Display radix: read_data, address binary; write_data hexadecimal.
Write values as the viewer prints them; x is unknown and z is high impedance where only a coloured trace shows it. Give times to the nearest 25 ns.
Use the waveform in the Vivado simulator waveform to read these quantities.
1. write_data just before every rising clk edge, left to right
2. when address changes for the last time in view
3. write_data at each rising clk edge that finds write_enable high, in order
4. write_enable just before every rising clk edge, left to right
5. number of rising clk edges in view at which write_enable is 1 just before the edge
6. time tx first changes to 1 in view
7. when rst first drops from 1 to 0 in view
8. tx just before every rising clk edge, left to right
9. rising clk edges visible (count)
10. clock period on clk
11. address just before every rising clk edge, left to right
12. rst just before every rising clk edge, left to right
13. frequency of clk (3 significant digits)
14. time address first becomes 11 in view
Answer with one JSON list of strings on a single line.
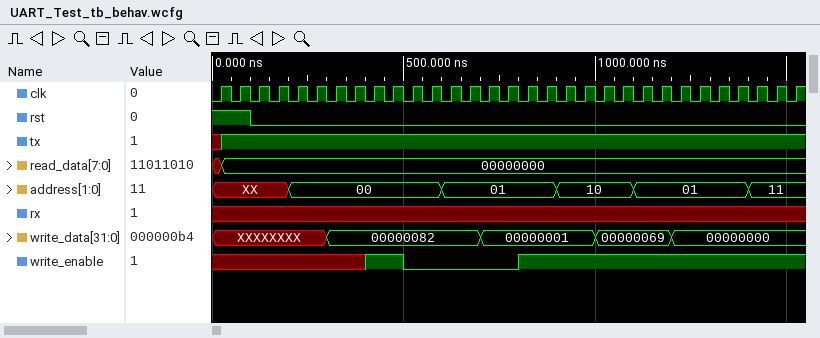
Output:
["XXXXXXXX, XXXXXXXX, XXXXXXXX, XXXXXXXX, XXXXXXXX, XXXXXXXX, 00000082, 00000082, 00000082, 00000082, 00000082, 00000082, 00000082, 00000082, 00000001, 00000001, 00000001, 00000001, 00000001, 00000001, 00000069, 00000069, 00000069, 00000069, 00000000, 00000000, 00000000, 00000000, 00000000, 00000000, 00000000", "1400 ns", "00000082, 00000082, 00000001, 00000001, 00000001, 00000001, 00000069, 00000069, 00000069, 00000069, 00000000, 00000000, 00000000, 00000000, 00000000, 00000000, 00000000", "x x x x x x x x 1 1 0 0 0 0 0 0 1 1 1 1 1 1 1 1 1 1 1 1 1 1 1", "17", "25 ns", "100 ns", "x 1 1 1 1 1 1 1 1 1 1 1 1 1 1 1 1 1 1 1 1 1 1 1 1 1 1 1 1 1 1", "31", "50 ns", "XX, XX, XX, XX, 00, 00, 00, 00, 00, 00, 00, 00, 01, 01, 01, 01, 01, 01, 10, 10, 10, 10, 01, 01, 01, 01, 01, 01, 11, 11, 11", "1 1 0 0 0 0 0 0 0 0 0 0 0 0 0 0 0 0 0 0 0 0 0 0 0 0 0 0 0 0 0", "20.0 MHz", "1400 ns"]
